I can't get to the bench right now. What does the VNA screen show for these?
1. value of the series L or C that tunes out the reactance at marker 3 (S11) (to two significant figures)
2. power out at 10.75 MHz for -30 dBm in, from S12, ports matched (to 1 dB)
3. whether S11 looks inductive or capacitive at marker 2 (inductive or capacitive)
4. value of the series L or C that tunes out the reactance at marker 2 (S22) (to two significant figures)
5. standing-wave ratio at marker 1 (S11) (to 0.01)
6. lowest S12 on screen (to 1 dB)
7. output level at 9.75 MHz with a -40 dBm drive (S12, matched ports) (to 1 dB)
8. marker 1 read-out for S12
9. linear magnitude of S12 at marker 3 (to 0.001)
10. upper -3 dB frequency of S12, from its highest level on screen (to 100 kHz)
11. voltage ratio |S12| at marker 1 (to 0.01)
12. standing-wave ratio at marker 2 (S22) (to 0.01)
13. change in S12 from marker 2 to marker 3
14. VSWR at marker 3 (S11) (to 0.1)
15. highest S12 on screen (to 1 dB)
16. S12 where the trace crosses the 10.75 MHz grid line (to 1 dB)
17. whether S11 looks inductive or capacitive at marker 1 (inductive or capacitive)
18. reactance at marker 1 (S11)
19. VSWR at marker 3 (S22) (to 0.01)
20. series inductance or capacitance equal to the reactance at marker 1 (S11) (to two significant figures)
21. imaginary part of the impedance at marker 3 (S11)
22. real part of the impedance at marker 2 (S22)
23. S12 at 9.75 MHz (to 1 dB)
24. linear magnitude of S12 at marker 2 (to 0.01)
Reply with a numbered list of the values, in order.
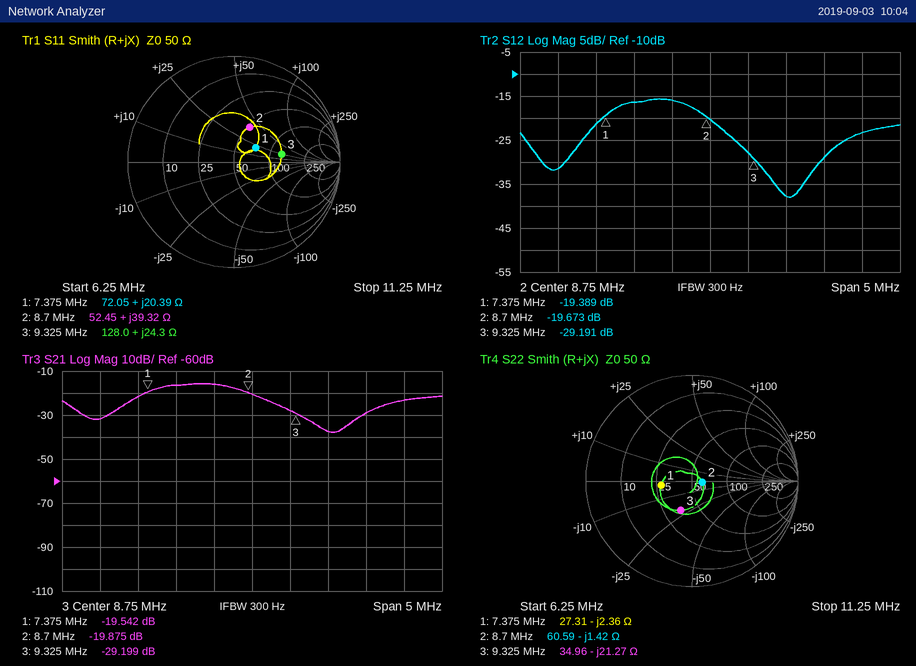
1. 700 pF
2. -53 dBm
3. inductive
4. 26 nH
5. 1.64
6. -38 dB
7. -78 dBm
8. -19.389 dB
9. 0.035
10. 8.6 MHz
11. 0.11
12. 1.21
13. -9.518 dB
14. 2.7
15. -16 dB
16. -23 dB
17. inductive
18. +20.39 Ω
19. 1.85
20. 440 nH
21. +24.3 Ω
22. 60.59 Ω
23. -38 dB
24. 0.10
